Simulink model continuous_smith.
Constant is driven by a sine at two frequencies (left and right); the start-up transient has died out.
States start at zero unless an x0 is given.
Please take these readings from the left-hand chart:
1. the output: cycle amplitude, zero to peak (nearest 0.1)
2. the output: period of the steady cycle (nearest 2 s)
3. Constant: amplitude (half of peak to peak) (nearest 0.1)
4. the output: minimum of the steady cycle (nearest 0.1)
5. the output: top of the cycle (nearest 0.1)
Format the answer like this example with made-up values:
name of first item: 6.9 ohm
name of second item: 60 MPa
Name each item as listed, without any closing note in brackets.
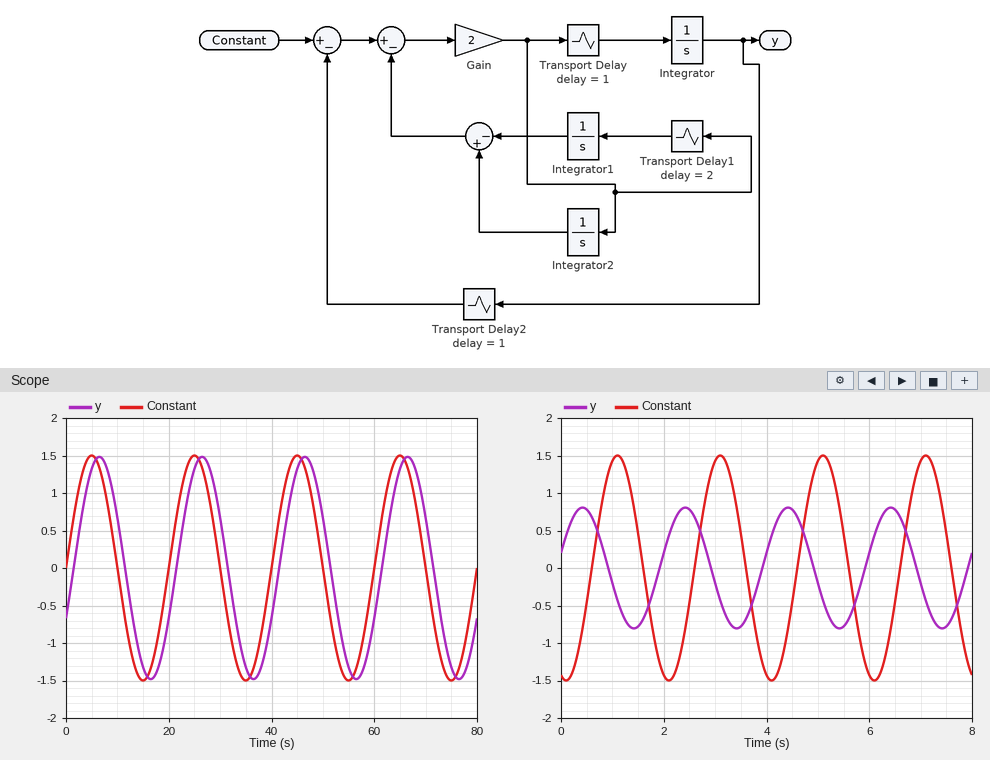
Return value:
the output: cycle amplitude, zero to peak: 1.5
the output: period of the steady cycle: 20 s
Constant: amplitude (half of peak to peak): 1.5
the output: minimum of the steady cycle: -1.5
the output: top of the cycle: 1.5
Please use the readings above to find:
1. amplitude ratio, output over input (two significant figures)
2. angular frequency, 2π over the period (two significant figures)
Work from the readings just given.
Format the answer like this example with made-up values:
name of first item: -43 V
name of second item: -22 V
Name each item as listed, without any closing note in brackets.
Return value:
amplitude ratio, output over input: 1.0
angular frequency, 2π over the period: 0.31 rad/s
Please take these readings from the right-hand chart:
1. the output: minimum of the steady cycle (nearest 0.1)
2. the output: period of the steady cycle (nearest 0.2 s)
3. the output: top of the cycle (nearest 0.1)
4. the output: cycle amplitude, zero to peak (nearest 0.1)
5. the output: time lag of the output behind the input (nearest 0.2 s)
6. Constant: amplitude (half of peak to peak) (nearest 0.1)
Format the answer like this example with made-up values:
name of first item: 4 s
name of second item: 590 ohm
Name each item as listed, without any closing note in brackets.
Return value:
the output: minimum of the steady cycle: -0.8
the output: period of the steady cycle: 2.0 s
the output: top of the cycle: 0.8
the output: cycle amplitude, zero to peak: 0.8
the output: time lag of the output behind the input: 1.4 s
Constant: amplitude (half of peak to peak): 1.5
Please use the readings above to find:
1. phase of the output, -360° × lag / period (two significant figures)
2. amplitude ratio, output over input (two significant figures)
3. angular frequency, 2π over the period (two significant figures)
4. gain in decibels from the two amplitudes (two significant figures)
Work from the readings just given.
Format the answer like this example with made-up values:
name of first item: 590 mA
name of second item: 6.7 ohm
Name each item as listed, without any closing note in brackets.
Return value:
phase of the output, -360° × lag / period: -250°
amplitude ratio, output over input: 0.53
angular frequency, 2π over the period: 3.1 rad/s
gain in decibels from the two amplitudes: -5.5 dB
